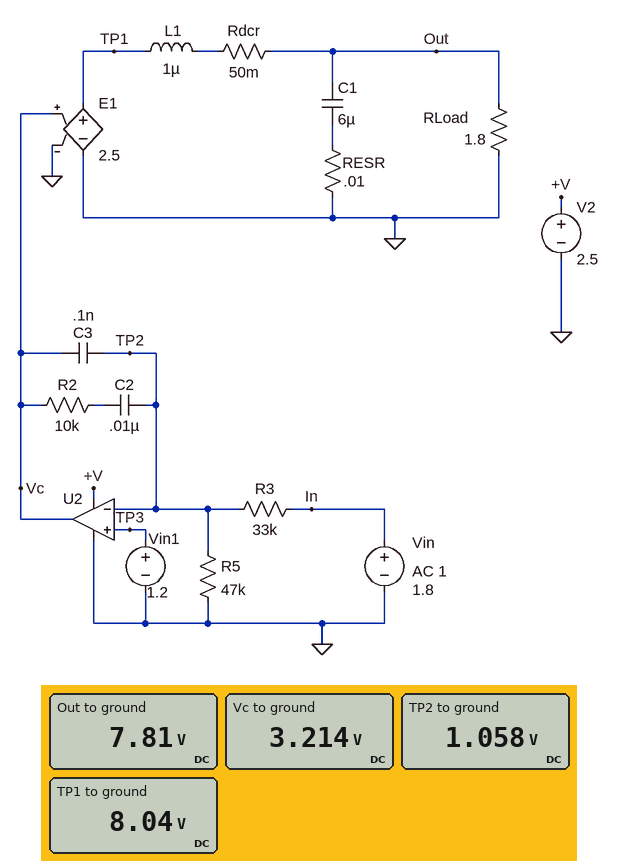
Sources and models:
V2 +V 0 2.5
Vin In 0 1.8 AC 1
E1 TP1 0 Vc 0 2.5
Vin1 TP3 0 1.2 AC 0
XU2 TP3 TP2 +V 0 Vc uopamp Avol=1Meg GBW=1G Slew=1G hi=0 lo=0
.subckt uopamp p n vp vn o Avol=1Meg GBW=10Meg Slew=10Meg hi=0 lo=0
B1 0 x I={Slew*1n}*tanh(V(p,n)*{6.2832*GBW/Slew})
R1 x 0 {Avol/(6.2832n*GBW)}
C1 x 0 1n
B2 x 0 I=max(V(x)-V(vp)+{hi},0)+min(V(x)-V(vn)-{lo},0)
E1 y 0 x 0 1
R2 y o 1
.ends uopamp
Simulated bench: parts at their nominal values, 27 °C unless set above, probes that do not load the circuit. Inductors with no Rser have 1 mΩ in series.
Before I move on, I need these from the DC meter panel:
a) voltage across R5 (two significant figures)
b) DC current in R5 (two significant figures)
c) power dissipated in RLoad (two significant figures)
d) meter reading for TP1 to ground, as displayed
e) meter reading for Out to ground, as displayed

1.1 V
23 µA
34 W
8.04 V
7.81 V
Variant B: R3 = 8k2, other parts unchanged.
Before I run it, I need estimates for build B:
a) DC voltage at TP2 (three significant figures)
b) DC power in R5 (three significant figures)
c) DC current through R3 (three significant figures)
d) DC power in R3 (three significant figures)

1.53 V
50.0 µW
32.6 µA
8.72 µW
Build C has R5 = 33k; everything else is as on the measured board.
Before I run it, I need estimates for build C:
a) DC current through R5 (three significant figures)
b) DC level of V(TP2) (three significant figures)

27.3 µA
900 mV
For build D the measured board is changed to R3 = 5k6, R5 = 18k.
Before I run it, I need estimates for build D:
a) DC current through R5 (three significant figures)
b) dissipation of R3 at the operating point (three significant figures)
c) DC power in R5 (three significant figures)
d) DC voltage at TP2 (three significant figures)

76.3 µA
32.6 µW
105 µW
1.37 V
